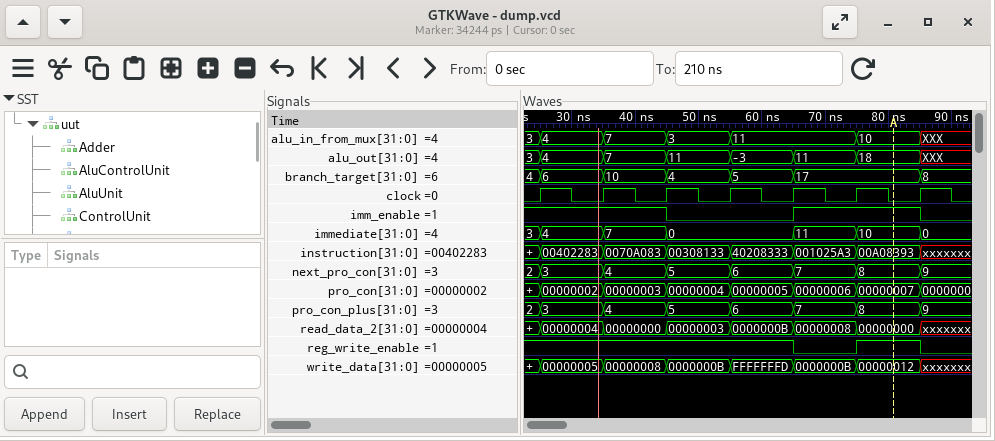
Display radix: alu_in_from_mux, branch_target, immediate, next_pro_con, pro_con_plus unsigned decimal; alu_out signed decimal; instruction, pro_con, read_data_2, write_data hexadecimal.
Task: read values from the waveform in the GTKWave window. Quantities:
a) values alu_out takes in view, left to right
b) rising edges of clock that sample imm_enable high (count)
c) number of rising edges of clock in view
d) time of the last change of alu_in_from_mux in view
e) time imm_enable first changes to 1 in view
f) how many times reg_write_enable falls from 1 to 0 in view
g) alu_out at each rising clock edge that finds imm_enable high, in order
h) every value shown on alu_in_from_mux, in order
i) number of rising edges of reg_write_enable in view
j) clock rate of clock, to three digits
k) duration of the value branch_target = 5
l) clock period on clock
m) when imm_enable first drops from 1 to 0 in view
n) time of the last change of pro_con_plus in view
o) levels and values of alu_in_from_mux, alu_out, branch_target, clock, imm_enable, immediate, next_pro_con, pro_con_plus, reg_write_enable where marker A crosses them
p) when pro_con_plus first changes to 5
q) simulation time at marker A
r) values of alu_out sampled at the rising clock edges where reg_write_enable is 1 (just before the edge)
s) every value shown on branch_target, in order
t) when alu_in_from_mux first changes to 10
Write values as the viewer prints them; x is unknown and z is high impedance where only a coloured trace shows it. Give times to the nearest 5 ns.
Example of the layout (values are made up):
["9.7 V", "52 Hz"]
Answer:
["3, 4, 7, 11, -3, 11, 18, XXX", "5", "7", "85 ns", "65 ns", "2", "3, 4, 7, 11, 18", "3, 4, 7, 3, 11, 10, XXX", "1", "100 MHz", "10 ns", "10 ns", "45 ns", "85 ns", "alu_in_from_mux=10, alu_out=18, branch_target=17, clock=0, imm_enable=1, immediate=10, next_pro_con=8, pro_con_plus=8, reg_write_enable=1", "45 ns", "80 ns", "3, 4, 7, 11, -3, 18", "4, 6, 10, 4, 5, 17, 8", "75 ns"]
